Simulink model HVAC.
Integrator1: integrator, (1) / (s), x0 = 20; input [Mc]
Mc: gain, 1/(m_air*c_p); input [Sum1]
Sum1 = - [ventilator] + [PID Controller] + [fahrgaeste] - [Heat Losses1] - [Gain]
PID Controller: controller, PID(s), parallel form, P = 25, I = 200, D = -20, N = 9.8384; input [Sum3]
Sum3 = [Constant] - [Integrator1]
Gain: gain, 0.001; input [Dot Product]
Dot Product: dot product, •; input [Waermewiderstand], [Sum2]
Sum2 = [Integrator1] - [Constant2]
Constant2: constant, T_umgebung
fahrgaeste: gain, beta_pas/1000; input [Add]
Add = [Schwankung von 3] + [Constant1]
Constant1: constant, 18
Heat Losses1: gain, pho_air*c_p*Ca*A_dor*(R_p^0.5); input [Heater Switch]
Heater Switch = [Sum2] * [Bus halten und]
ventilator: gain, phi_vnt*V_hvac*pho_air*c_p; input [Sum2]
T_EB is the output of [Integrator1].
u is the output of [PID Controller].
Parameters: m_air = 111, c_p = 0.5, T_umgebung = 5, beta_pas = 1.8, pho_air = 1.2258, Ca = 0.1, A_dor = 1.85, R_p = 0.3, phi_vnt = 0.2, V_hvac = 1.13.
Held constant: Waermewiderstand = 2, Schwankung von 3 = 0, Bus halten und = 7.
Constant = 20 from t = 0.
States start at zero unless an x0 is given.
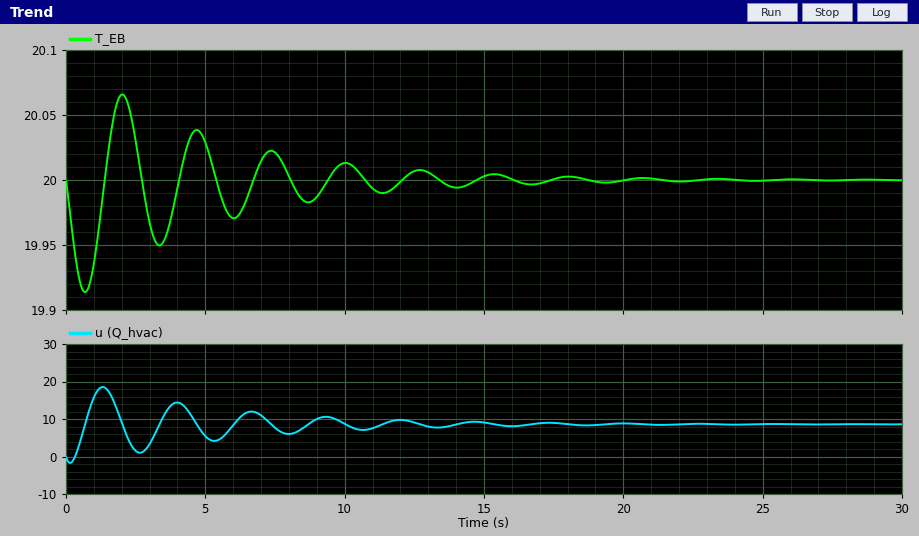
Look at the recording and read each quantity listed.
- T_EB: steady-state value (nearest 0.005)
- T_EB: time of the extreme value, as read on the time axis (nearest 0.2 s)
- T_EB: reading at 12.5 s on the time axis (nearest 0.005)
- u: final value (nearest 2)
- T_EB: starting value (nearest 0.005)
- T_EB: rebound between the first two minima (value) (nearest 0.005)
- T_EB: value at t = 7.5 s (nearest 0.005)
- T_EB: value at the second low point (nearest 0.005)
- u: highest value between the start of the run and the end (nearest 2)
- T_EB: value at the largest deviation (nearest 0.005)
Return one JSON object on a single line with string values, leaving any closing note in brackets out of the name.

{"T_EB: steady-state value": "20.000", "T_EB: time of the extreme value, as read on the time axis": "0.6 s", "T_EB: reading at 12.5 s on the time axis": "20.005", "u: final value": "8", "T_EB: starting value": "20.000", "T_EB: rebound between the first two minima (value)": "20.065", "T_EB: value at t = 7.5 s": "20.020", "T_EB: value at the second low point": "19.950", "u: highest value between the start of the run and the end": "18", "T_EB: value at the largest deviation": "19.915"}
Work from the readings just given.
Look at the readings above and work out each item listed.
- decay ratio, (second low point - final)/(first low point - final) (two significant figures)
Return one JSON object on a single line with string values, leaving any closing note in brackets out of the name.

{"decay ratio, (second low point - final)/(first low point - final)": "0.59"}
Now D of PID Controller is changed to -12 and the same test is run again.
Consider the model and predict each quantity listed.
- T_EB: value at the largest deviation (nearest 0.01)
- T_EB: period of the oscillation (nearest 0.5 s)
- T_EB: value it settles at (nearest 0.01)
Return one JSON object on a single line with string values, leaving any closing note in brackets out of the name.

{"T_EB: value at the largest deviation": "19.92", "T_EB: period of the oscillation": "3.0 s", "T_EB: value it settles at": "20.00"}
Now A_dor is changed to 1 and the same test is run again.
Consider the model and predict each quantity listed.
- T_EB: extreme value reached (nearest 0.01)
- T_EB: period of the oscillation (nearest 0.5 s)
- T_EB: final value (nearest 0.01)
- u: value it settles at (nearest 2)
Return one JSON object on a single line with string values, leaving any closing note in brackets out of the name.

{"T_EB: extreme value reached": "19.94", "T_EB: period of the oscillation": "2.5 s", "T_EB: final value": "20.00", "u: value it settles at": "6"}
